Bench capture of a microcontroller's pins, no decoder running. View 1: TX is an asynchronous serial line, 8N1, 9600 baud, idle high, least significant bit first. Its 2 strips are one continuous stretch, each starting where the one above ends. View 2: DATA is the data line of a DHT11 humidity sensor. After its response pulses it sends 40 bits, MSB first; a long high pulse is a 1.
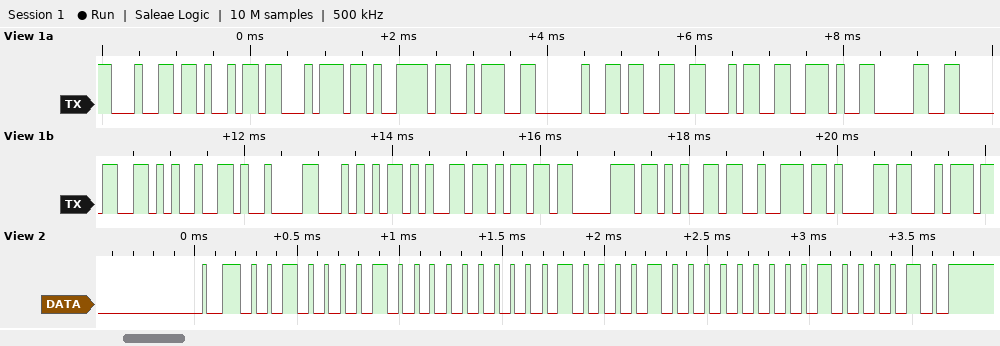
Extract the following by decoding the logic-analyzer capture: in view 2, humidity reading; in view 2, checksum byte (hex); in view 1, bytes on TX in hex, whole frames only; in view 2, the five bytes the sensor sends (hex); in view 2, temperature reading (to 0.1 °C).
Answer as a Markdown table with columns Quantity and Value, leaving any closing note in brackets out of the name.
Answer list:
| Quantity | Value |
|---|---|
| in view 2, humidity reading | 33 % |
| in view 2, checksum byte | 0x42 |
| in view 1, bytes on TX in hex, whole frames only | 64 69 74 79 3A 20 33 34 2E 30 30 25 09 54 65 6D 70 65 72 61 74 |
| in view 2, the five bytes the sensor sends | 21 00 21 00 42 |
| in view 2, temperature reading | 33.0 °C |
